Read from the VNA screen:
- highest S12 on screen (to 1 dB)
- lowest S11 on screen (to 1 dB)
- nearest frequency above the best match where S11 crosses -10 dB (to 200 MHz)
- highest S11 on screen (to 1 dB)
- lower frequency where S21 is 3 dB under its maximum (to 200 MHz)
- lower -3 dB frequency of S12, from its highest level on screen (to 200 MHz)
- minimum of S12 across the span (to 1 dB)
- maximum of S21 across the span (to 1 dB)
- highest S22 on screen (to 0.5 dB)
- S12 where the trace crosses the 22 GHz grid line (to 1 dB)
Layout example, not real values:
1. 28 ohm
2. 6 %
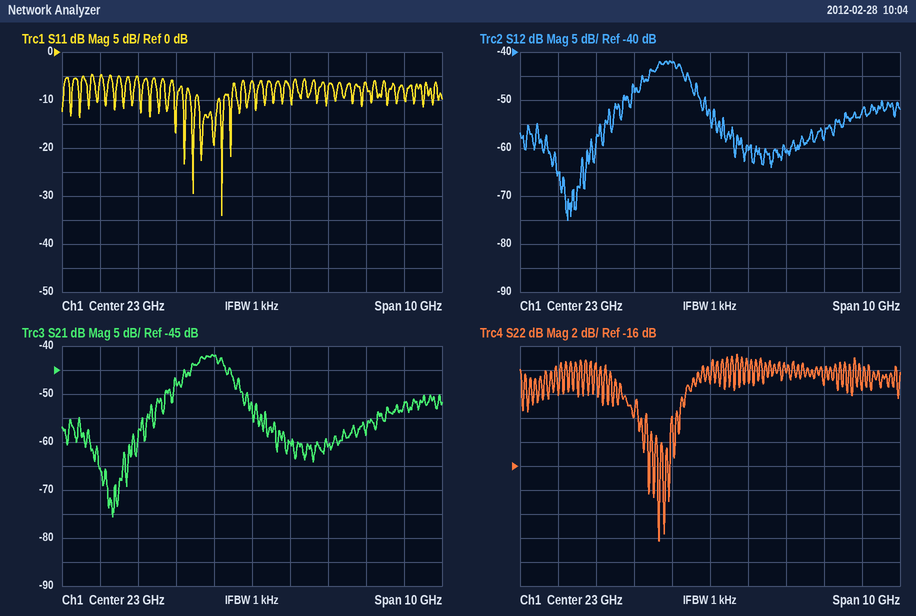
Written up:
1. -42 dB
2. -34 dB
3. 22.2 GHz
4. -5 dB
5. 21.4 GHz
6. 21.4 GHz
7. -75 dB
8. -42 dB
9. -6.5 dB
10. -42 dB
